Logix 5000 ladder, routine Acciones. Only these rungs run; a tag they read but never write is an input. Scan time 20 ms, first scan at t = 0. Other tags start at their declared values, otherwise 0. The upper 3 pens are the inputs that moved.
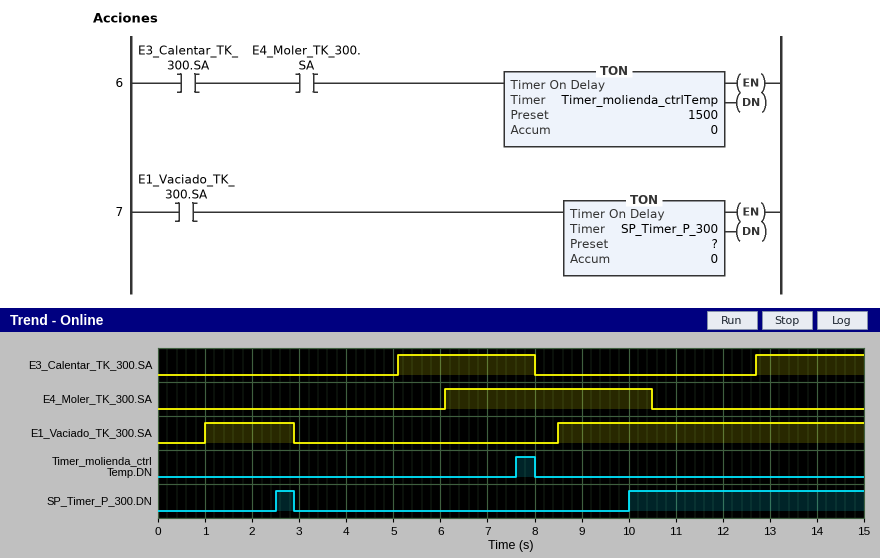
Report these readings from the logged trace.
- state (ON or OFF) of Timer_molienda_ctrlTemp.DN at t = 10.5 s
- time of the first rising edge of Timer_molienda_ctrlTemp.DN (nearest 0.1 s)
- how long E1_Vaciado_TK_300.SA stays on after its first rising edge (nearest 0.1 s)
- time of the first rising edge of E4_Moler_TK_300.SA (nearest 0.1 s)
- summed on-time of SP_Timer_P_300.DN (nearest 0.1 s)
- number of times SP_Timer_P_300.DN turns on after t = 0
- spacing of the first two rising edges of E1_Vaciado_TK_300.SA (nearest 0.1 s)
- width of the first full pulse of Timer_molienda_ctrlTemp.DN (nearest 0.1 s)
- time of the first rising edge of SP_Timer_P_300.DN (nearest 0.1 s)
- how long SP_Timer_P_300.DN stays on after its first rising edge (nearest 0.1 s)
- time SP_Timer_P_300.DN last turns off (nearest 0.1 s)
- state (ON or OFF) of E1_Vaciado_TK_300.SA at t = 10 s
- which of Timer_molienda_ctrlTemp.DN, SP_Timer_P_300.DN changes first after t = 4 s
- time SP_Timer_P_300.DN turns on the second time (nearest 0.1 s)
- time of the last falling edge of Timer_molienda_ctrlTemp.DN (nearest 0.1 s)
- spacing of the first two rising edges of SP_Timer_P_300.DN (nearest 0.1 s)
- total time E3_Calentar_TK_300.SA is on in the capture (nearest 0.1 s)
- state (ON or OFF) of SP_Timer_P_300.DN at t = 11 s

OFF
7.6 s
1.9 s
6.1 s
5.4 s
2
7.5 s
0.4 s
2.5 s
0.4 s
2.9 s
ON
Timer_molienda_ctrlTemp.DN
10.0 s
8.0 s
7.5 s
5.2 s
ON
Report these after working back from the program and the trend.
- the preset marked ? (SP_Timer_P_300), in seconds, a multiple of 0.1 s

1.5 s
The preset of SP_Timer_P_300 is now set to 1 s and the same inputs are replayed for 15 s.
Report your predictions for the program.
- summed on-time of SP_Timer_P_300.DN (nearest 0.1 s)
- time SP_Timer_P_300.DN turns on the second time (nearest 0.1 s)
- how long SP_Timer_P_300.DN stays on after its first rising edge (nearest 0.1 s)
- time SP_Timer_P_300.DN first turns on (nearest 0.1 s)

6.4 s
9.5 s
0.9 s
2.0 s
